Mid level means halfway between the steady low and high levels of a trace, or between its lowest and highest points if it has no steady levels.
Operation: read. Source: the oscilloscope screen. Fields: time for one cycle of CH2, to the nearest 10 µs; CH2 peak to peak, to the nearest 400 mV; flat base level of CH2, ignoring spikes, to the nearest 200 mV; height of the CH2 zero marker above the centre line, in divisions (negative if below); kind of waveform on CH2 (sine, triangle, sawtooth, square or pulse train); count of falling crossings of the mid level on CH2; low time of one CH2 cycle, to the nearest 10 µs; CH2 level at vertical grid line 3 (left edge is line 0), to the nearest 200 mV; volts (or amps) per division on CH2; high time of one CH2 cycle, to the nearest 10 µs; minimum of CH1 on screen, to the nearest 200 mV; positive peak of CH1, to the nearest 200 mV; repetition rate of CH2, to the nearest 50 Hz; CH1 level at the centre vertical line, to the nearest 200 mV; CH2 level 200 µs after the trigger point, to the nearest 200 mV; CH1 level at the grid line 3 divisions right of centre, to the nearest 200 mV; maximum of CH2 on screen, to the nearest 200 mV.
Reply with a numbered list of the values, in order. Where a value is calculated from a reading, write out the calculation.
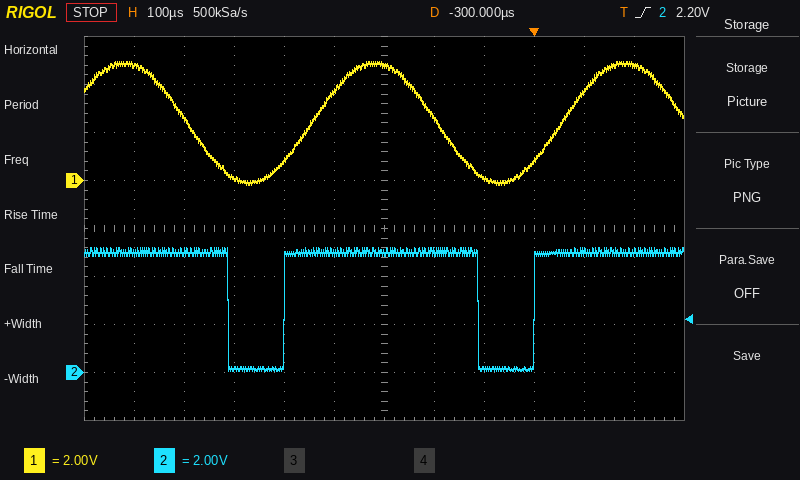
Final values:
1. 500 µs
2. 5.2 V
3. 200 mV
4. -3.0 div
5. pulse train
6. 2
7. 110 µs
8. 200 mV
9. 2 V
10. 390 µs
11. -200 mV
12. 5.0 V
13. 1 / 500 µs ≈ 2.00 kHz
14. 4.8 V
15. 5.0 V
16. 800 mV
17. 5.2 V
